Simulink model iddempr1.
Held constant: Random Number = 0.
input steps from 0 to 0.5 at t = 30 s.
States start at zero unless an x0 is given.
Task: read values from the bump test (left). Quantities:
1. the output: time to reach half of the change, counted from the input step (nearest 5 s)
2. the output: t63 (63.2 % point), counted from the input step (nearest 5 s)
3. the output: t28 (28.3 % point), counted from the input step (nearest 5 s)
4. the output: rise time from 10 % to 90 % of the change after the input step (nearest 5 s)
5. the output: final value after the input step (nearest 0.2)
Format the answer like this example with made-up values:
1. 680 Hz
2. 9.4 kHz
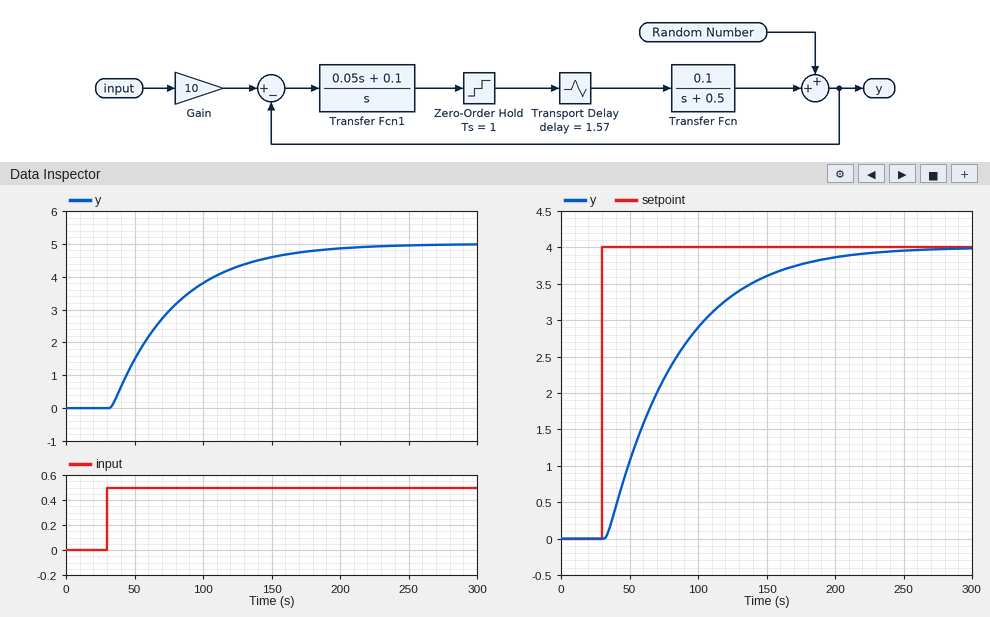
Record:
1. 35 s
2. 50 s
3. 20 s
4. 100 s
5. 5.0
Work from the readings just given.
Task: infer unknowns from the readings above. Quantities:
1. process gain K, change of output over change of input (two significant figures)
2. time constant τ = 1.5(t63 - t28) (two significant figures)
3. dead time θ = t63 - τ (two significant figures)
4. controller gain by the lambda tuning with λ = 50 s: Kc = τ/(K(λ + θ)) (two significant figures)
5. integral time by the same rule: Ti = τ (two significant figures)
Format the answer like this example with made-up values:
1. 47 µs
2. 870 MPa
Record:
1. 10
2. 45 s
3. 5.0 s
4. 0.082
5. 45 s
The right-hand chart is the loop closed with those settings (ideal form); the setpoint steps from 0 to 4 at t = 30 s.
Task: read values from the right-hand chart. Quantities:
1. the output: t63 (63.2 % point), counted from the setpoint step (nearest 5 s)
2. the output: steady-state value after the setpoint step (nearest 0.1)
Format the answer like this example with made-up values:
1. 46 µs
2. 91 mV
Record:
1. 55 s
2. 4.0
